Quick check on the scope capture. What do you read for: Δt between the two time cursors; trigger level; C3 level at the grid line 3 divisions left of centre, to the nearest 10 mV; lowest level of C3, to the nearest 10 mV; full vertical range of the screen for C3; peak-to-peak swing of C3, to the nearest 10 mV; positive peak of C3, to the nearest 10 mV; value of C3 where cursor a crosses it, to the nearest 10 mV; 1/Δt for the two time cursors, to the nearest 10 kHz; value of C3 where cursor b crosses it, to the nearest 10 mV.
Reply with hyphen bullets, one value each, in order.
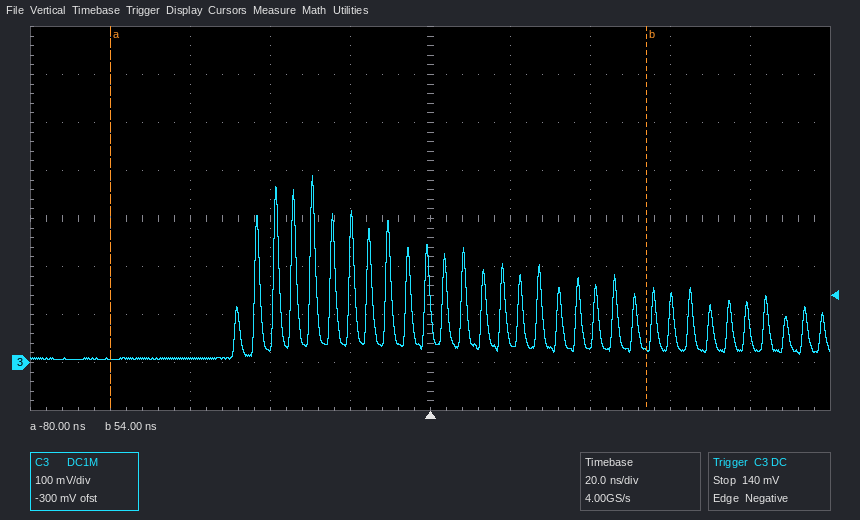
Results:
- 134 ns
- 140 mV
- 10 mV
- 10 mV
- 800 mV
- 380 mV
- 390 mV
- 10 mV
- 7.46 MHz
- 30 mV
